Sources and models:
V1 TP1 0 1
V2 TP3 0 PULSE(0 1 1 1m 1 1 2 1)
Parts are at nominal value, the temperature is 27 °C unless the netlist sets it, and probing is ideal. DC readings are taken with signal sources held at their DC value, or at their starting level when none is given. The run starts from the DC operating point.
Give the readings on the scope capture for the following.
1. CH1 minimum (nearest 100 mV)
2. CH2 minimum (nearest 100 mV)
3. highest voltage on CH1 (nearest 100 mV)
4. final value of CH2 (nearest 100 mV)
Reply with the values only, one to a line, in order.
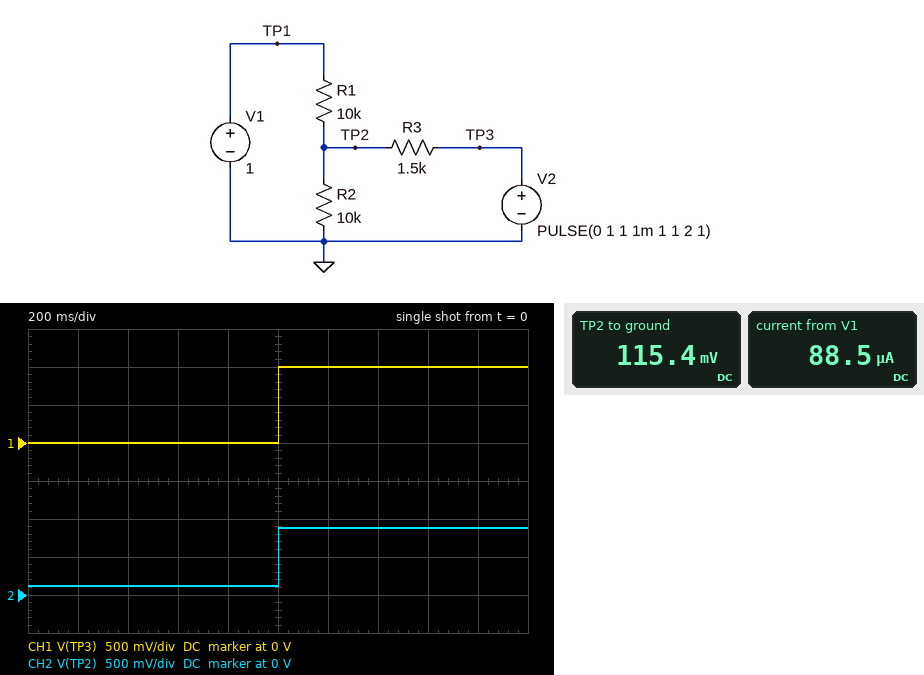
0 V
100 mV
1.0 V
900 mV
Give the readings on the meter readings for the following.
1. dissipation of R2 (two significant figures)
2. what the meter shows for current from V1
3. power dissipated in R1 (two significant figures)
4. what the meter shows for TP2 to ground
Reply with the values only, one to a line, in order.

1.3 µW
88.5 µA
78 µW
115.4 mV
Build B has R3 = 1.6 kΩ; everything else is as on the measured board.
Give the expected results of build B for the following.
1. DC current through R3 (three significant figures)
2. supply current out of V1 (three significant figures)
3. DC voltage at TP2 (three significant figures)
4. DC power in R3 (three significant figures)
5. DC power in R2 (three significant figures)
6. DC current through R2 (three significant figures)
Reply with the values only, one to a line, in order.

75.8 µA
87.9 µA
121 mV
9.18 µW
1.47 µW
12.1 µA
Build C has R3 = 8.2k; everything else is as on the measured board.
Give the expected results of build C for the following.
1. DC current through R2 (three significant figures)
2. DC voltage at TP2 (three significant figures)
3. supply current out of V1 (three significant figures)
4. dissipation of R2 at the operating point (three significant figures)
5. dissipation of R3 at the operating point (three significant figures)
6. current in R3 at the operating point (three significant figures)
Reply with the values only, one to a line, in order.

31.1 µA
311 mV
68.9 µA
9.65 µW
11.8 µW
37.9 µA
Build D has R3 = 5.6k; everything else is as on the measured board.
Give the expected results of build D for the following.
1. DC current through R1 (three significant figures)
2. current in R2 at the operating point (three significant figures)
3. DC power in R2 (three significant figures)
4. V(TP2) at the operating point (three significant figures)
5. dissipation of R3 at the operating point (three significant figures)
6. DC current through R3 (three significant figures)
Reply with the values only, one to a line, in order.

73.6 µA
26.4 µA
6.98 µW
264 mV
12.5 µW
47.2 µA
